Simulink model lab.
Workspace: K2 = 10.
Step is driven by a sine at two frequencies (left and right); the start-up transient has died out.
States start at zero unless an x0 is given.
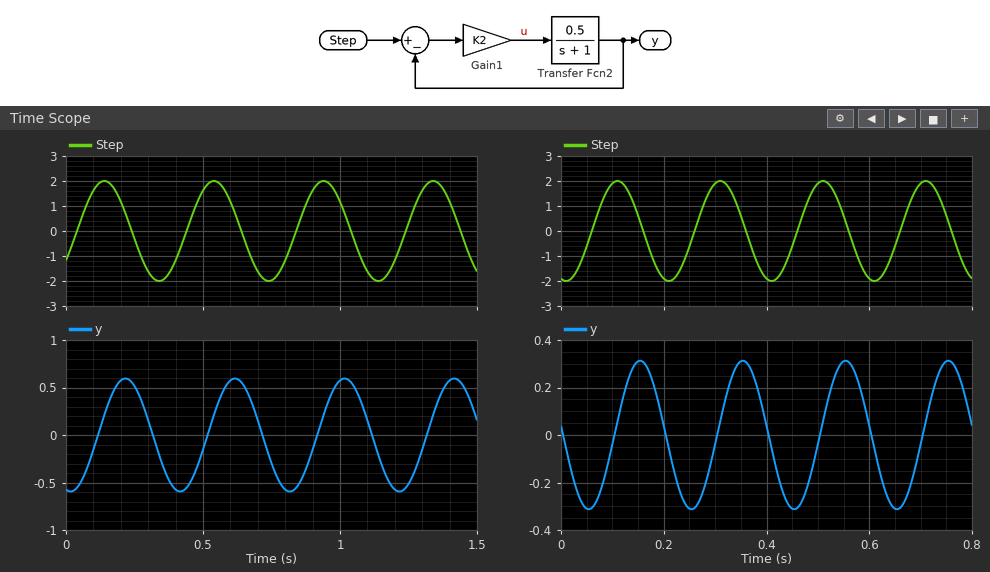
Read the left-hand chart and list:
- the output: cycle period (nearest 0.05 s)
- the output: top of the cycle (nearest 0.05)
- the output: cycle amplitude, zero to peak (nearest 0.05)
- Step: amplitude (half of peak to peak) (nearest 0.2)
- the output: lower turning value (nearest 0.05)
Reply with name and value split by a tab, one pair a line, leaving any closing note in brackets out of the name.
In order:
the output: cycle period	0.40 s
the output: top of the cycle	0.60
the output: cycle amplitude, zero to peak	0.60
Step: amplitude (half of peak to peak)	2.0
the output: lower turning value	-0.60
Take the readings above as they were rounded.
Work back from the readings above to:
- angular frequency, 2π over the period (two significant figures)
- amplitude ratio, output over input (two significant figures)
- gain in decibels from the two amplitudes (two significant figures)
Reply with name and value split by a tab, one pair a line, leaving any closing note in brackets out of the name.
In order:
angular frequency, 2π over the period	16 rad/s
amplitude ratio, output over input	0.30
gain in decibels from the two amplitudes	-10 dB
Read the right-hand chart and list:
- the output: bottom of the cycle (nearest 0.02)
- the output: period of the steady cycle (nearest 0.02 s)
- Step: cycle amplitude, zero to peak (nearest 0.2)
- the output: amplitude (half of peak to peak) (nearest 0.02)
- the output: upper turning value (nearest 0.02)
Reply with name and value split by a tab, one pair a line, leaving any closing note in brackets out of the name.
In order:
the output: bottom of the cycle	-0.32
the output: period of the steady cycle	0.20 s
Step: cycle amplitude, zero to peak	2.0
the output: amplitude (half of peak to peak)	0.32
the output: upper turning value	0.32
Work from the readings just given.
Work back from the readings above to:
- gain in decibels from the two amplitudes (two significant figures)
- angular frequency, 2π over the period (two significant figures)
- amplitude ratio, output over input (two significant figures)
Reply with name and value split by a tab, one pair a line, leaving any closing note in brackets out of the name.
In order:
gain in decibels from the two amplitudes	-16 dB
angular frequency, 2π over the period	31 rad/s
amplitude ratio, output over input	0.16
